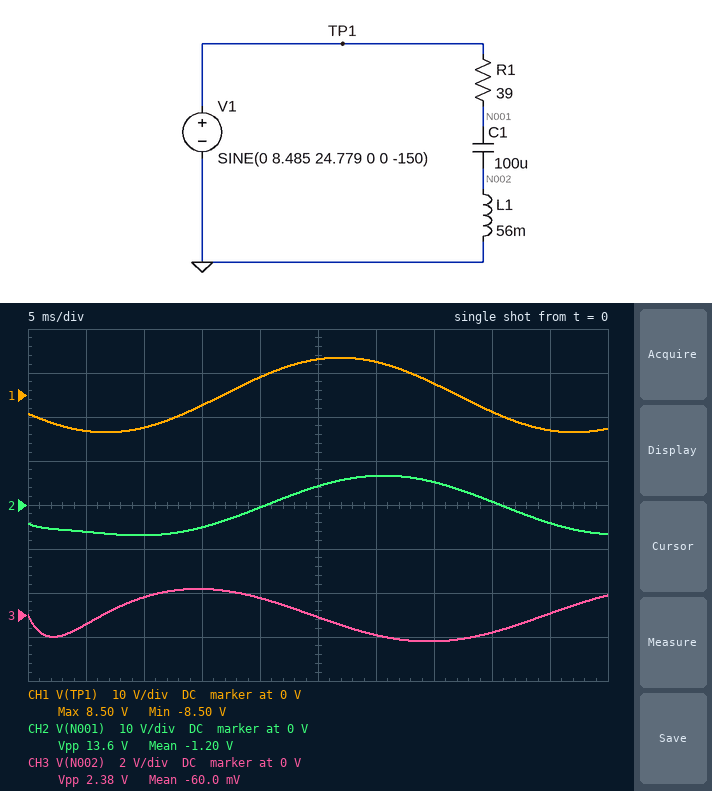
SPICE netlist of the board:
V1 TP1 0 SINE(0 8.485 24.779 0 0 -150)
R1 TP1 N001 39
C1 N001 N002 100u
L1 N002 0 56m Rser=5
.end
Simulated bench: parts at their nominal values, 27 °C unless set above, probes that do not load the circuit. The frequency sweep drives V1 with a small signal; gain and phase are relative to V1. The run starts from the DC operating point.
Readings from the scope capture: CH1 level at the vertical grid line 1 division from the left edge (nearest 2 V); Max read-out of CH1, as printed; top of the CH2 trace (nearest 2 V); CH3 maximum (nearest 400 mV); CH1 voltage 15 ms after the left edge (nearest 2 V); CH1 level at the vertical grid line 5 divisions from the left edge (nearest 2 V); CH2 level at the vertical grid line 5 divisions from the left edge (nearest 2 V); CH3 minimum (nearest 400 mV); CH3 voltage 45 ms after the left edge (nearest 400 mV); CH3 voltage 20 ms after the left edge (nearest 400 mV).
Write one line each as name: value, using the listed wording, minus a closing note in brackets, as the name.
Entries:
CH1 level at the vertical grid line 1 division from the left edge: -8 V
Max read-out of CH1, as printed: 8.50 V
top of the CH2 trace: 6 V
CH3 maximum: 1.2 V
CH1 voltage 15 ms after the left edge: -2 V
CH1 level at the vertical grid line 5 divisions from the left edge: 8 V
CH2 level at the vertical grid line 5 divisions from the left edge: 4 V
CH3 minimum: -1.2 V
CH3 voltage 45 ms after the left edge: 0 V
CH3 voltage 20 ms after the left edge: 800 mV
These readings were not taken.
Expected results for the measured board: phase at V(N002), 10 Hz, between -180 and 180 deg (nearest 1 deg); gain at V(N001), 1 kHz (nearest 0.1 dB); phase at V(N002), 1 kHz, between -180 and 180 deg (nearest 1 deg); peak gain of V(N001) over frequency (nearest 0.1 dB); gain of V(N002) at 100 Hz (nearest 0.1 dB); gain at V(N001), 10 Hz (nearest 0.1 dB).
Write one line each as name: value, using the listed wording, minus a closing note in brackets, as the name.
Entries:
phase at V(N002), 10 Hz, between -180 and 180 deg: 109 deg
gain at V(N001), 1 kHz: -0.1 dB
phase at V(N002), 1 kHz, between -180 and 180 deg: 6 deg
peak gain of V(N001) over frequency: 0 dB
gain of V(N002) at 100 Hz: -2.6 dB
gain at V(N001), 10 Hz: -0.3 dB
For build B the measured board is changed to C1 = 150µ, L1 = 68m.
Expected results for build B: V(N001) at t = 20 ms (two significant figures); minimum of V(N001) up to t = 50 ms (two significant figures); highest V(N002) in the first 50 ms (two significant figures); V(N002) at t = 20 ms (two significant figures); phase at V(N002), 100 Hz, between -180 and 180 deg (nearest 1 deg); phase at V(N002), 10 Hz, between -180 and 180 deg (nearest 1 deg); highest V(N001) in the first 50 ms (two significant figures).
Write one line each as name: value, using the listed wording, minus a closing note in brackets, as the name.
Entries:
V(N001) at t = 20 ms: -1.6 V
minimum of V(N001) up to t = 50 ms: -6.2 V
highest V(N002) in the first 50 ms: 1.7 V
V(N002) at t = 20 ms: 1.4 V
phase at V(N002), 100 Hz, between -180 and 180 deg: 47 deg
phase at V(N002), 10 Hz, between -180 and 180 deg: 107 deg
highest V(N001) in the first 50 ms: 5.1 V
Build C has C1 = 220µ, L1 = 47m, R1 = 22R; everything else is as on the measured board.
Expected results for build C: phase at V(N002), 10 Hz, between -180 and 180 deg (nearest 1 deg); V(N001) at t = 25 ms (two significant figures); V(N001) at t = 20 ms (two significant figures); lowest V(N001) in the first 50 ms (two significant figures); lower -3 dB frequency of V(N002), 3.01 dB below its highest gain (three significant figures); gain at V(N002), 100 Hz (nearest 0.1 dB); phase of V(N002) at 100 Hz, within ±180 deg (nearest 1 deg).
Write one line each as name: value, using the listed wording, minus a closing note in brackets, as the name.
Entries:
phase at V(N002), 10 Hz, between -180 and 180 deg: 99 deg
V(N001) at t = 25 ms: 3.1 V
V(N001) at t = 20 ms: -940 mV
lowest V(N001) in the first 50 ms: -6.4 V
lower -3 dB frequency of V(N002), 3.01 dB below its highest gain: 65.5 Hz
gain at V(N002), 100 Hz: -1.4 dB
phase of V(N002) at 100 Hz, within ±180 deg: 41 deg
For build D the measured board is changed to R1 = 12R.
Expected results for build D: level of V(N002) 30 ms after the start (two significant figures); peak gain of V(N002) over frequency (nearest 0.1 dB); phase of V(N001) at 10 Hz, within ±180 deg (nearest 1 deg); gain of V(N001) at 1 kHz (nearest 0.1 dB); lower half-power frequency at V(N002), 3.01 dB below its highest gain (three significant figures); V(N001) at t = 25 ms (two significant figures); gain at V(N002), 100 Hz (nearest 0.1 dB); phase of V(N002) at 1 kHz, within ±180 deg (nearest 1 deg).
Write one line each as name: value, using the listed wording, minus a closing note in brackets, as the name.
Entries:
level of V(N002) 30 ms after the start: -1.4 V
peak gain of V(N002) over frequency: 3.6 dB
phase of V(N001) at 10 Hz, within ±180 deg: -4 deg
gain of V(N001) at 1 kHz: 0 dB
lower half-power frequency at V(N002), 3.01 dB below its highest gain: 56.2 Hz
V(N001) at t = 25 ms: 7.2 V
gain at V(N002), 100 Hz: 2.8 dB
phase of V(N002) at 1 kHz, within ±180 deg: 2 deg
